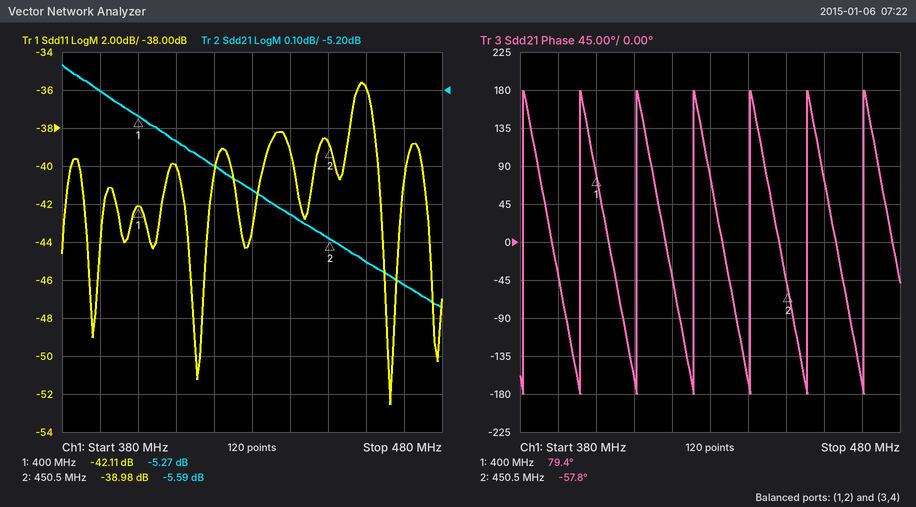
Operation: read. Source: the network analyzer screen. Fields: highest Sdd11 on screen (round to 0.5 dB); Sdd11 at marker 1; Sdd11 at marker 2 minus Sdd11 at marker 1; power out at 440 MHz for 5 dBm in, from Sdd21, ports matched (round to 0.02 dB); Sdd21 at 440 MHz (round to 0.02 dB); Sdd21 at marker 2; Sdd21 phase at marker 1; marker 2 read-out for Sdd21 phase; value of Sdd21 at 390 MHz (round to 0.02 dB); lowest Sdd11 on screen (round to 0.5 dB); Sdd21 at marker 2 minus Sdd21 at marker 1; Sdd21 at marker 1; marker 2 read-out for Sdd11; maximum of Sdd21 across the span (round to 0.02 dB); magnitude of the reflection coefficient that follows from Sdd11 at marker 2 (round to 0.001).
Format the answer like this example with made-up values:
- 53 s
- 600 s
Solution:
- -35.5 dB
- -42.11 dB
- 3.13 dB
- -0.52 dBm
- -5.52 dB
- -5.59 dB
- 79.4°
- -57.8°
- -5.20 dB
- -52.5 dB
- -0.32 dB
- -5.27 dB
- -38.98 dB
- -5.14 dB
- 0.011
